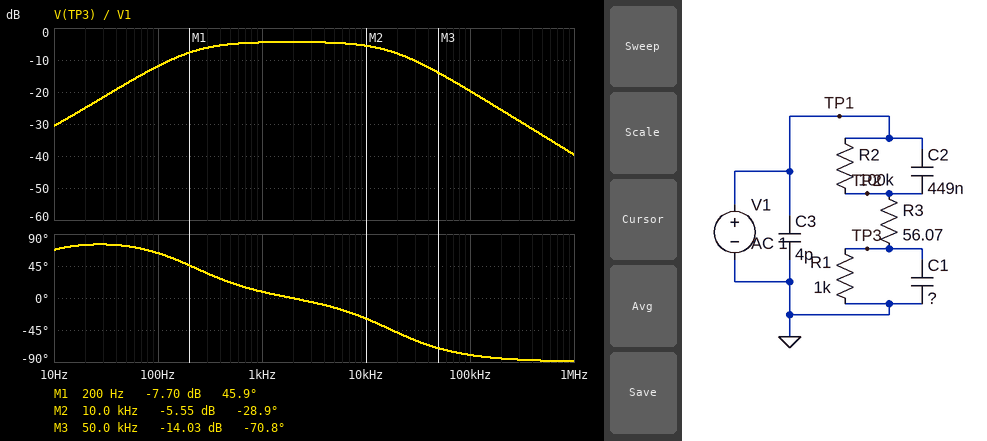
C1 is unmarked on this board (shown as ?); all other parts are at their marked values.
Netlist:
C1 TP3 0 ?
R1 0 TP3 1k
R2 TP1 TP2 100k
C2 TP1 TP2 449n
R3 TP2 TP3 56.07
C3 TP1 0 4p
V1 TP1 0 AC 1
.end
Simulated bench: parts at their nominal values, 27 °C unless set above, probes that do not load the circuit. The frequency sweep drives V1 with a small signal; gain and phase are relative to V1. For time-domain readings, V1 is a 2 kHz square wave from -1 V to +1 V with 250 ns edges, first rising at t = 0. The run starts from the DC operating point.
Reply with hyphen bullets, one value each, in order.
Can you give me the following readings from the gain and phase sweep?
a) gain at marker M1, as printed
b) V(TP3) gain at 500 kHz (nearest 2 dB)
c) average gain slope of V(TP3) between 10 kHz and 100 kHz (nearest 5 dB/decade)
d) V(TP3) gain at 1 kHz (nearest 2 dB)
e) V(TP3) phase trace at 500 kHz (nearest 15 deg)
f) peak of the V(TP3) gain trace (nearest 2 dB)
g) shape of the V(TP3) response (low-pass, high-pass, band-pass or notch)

- -7.70 dB
- -34 dB
- -15 dB/decade
- -4 dB
- -90 deg
- -4 dB
- band-pass
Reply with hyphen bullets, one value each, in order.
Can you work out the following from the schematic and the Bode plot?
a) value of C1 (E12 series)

- 270 nF
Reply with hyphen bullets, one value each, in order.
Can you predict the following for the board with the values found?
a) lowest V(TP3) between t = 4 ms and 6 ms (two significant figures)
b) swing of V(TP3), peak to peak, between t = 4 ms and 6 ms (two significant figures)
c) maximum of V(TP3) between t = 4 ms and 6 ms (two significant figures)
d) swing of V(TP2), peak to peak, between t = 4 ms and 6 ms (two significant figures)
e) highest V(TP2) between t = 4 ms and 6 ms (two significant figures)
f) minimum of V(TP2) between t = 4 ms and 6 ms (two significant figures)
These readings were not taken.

- -670 mV
- 1.3 V
- 670 mV
- 2.9 V
- 1.5 V
- -1.5 V
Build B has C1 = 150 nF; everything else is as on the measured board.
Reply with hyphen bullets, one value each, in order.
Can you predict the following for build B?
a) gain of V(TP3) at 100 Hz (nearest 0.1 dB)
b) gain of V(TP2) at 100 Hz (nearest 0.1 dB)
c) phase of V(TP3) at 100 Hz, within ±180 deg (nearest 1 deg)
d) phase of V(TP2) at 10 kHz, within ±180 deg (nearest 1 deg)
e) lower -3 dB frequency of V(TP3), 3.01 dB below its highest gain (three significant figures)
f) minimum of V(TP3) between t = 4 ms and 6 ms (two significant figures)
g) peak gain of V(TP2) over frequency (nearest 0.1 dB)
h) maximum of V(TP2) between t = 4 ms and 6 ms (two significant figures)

- -11.7 dB
- -11.2 dB
- 67 deg
- 7 deg
- 255 Hz
- -830 mV
- 0 dB
- 1.4 V
